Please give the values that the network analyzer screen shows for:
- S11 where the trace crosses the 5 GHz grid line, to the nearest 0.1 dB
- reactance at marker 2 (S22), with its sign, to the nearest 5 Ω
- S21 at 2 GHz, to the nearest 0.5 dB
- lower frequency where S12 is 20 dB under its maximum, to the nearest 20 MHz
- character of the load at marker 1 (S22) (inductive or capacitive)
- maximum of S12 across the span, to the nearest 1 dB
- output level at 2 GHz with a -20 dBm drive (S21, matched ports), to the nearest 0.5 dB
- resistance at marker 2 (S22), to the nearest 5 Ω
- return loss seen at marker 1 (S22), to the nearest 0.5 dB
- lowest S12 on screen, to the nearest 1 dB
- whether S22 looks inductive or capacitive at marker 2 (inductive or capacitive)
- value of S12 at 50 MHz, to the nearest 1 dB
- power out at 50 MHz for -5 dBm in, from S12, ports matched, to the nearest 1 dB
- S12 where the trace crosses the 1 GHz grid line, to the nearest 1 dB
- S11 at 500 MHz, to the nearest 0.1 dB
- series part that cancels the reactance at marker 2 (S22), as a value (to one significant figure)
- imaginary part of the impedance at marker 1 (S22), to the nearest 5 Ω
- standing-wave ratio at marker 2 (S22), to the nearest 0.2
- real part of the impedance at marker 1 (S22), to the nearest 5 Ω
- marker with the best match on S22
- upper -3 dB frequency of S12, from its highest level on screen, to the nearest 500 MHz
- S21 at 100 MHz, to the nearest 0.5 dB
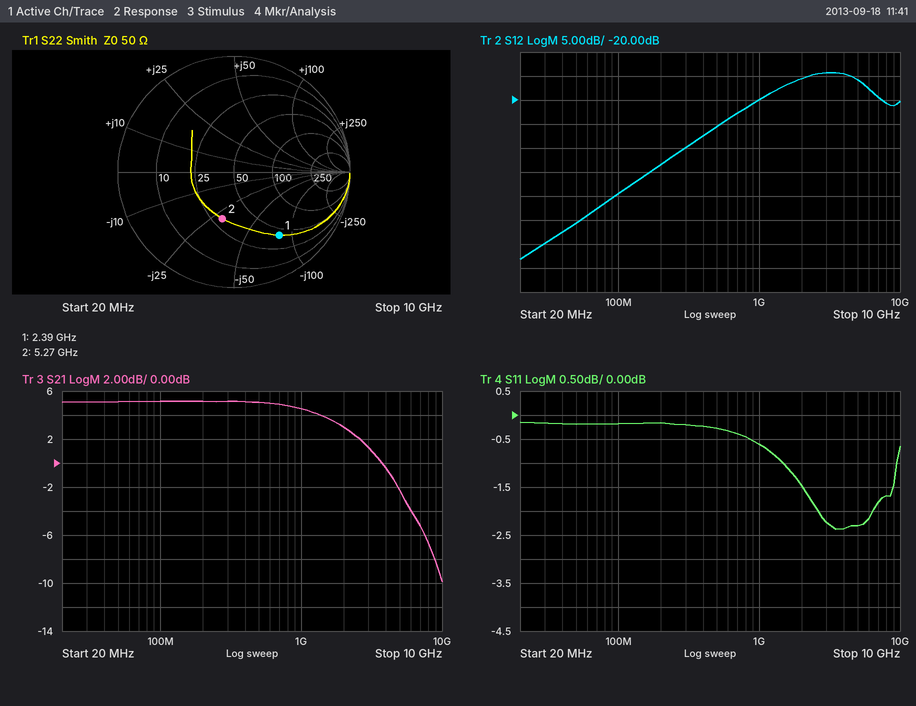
-2.3 dB
-30 Ω
3.0 dB
180 MHz
capacitive
-14 dB
-17.0 dBm
30 Ω
3.5 dB
-53 dB
capacitive
-46 dB
-51 dBm
-20 dB
-0.3 dB
900 pH
-80 Ω
2.4
40 Ω
marker 2
6.0 GHz
5.0 dB
